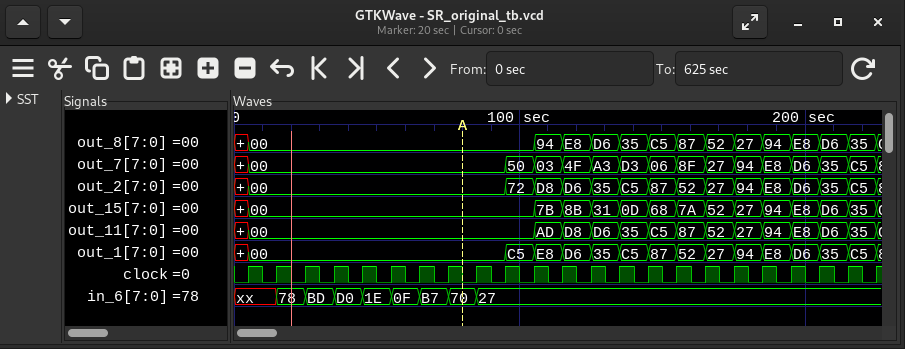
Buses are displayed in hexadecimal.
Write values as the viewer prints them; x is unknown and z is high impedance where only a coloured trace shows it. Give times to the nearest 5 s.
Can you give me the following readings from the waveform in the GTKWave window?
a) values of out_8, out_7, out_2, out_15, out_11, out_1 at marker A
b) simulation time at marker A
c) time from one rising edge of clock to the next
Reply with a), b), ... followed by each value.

a) out_8=00, out_7=00, out_2=00, out_15=00, out_11=00, out_1=00
b) 80 s
c) 10 s
